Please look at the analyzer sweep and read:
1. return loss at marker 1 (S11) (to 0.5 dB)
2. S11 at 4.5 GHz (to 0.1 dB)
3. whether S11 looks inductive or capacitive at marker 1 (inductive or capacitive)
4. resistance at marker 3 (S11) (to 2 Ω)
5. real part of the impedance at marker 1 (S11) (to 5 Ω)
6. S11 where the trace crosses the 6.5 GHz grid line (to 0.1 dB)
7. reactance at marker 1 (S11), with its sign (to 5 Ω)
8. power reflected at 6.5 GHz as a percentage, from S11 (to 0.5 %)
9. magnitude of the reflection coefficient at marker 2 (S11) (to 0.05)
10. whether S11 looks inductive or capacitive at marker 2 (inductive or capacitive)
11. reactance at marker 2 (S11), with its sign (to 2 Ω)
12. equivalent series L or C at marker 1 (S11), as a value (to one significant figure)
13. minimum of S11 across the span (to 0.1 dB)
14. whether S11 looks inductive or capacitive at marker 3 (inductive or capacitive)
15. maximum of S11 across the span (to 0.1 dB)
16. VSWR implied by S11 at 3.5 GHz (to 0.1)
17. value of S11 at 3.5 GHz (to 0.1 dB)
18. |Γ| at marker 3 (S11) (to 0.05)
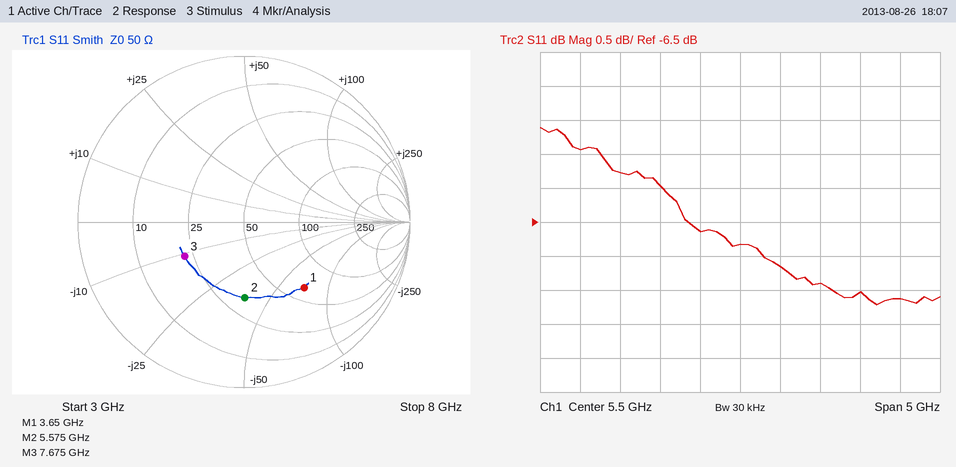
5.5 dB
-6.0 dB
capacitive
22 Ω
65 Ω
-7.4 dB
-70 Ω
18.0 %
0.45
capacitive
-38 Ω
600 fF
-7.7 dB
capacitive
-5.1 dB
3.3
-5.4 dB
0.40
